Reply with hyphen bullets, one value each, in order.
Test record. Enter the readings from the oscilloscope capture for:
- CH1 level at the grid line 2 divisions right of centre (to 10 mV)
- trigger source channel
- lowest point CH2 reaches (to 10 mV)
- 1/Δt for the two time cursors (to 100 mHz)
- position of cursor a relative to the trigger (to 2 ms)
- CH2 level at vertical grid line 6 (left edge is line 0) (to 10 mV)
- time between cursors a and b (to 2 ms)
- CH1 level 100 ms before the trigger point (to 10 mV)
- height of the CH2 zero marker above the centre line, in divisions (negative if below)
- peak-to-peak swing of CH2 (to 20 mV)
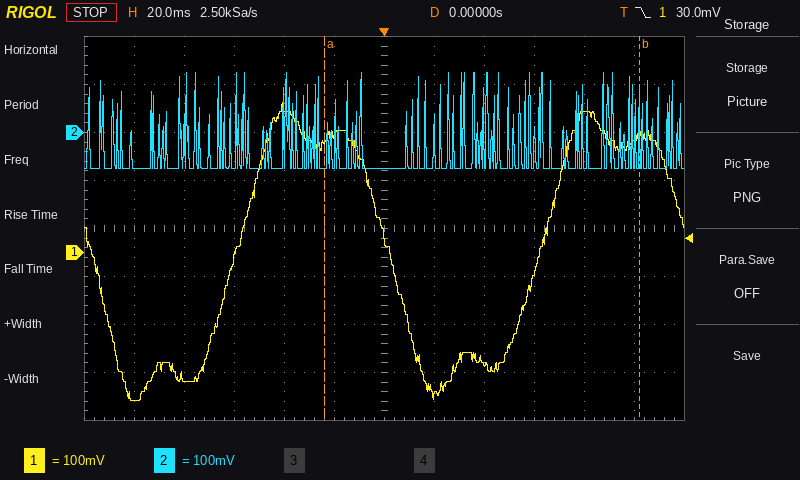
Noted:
- -230 mV
- CH1
- -80 mV
- 7.9 Hz
- -24 ms
- -80 mV
- 126 ms
- -310 mV
- +2.0 div
- 200 mV
